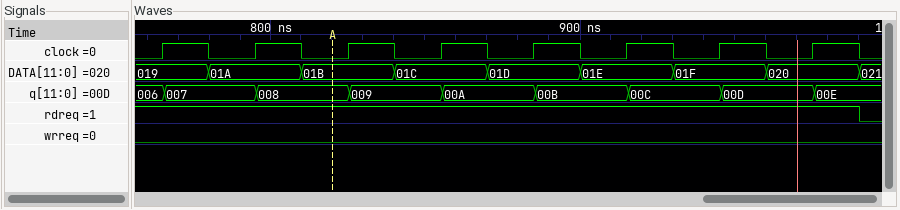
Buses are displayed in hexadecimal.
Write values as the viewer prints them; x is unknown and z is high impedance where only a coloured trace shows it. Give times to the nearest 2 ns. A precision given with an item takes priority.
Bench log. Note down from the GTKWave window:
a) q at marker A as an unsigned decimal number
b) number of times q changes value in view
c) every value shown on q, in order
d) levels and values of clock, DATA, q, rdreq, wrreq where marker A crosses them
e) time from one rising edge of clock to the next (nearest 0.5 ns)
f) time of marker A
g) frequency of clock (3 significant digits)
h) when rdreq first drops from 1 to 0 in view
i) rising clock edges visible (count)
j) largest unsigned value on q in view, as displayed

8
8
006, 007, 008, 009, 00A, 00B, 00C, 00D, 00E
clock=0, DATA=01B, q=008, rdreq=1, wrreq=0
30 ns
820 ns
33.3 MHz
990 ns
8
00E
